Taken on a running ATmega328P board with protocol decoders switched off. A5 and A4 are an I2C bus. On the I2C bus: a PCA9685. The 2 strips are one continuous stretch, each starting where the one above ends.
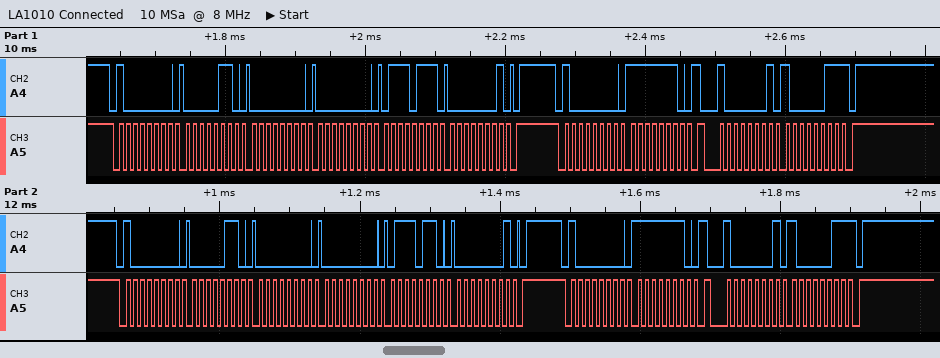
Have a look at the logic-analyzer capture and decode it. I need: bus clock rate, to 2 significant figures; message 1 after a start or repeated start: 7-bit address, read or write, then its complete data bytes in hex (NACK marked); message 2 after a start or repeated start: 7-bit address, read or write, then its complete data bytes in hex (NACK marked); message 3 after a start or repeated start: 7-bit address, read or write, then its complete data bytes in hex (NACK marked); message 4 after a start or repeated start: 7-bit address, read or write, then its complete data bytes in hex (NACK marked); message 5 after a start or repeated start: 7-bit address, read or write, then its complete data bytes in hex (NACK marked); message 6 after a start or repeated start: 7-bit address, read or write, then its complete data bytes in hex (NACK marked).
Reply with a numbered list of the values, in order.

1. 100 kHz
2. 0x40 write: 06 00 00 77 01
3. 0x40 write: FE
4. 0x40 read: 83 NACK
5. 0x40 write: 06 00 00 76 01
6. 0x40 write: FE
7. 0x40 read: 83 NACK
